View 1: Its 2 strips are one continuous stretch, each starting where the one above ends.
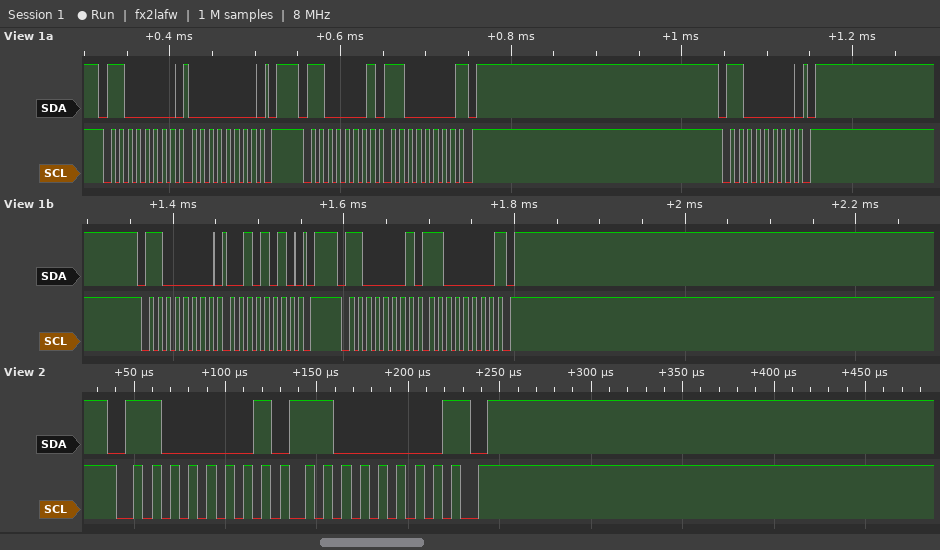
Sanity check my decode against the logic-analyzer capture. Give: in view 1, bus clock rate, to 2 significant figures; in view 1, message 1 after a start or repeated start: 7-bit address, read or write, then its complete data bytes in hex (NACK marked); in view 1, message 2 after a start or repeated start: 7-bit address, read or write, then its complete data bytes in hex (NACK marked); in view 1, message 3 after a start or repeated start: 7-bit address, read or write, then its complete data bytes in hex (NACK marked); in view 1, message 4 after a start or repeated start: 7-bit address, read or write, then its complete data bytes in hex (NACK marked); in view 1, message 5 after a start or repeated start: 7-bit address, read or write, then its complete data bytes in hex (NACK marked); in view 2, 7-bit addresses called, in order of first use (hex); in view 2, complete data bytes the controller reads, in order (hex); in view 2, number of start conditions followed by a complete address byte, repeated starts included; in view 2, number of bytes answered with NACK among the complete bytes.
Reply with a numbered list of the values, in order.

1. 100 kHz
2. 0x60 write: 00
3. 0x60 read: C0 NACK
4. 0x60 write
5. 0x60 write: 2A
6. 0x60 read: C0 NACK
7. 0x60
8. C0
9. 1
10. 1
